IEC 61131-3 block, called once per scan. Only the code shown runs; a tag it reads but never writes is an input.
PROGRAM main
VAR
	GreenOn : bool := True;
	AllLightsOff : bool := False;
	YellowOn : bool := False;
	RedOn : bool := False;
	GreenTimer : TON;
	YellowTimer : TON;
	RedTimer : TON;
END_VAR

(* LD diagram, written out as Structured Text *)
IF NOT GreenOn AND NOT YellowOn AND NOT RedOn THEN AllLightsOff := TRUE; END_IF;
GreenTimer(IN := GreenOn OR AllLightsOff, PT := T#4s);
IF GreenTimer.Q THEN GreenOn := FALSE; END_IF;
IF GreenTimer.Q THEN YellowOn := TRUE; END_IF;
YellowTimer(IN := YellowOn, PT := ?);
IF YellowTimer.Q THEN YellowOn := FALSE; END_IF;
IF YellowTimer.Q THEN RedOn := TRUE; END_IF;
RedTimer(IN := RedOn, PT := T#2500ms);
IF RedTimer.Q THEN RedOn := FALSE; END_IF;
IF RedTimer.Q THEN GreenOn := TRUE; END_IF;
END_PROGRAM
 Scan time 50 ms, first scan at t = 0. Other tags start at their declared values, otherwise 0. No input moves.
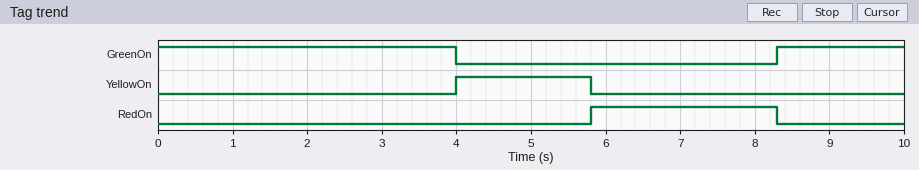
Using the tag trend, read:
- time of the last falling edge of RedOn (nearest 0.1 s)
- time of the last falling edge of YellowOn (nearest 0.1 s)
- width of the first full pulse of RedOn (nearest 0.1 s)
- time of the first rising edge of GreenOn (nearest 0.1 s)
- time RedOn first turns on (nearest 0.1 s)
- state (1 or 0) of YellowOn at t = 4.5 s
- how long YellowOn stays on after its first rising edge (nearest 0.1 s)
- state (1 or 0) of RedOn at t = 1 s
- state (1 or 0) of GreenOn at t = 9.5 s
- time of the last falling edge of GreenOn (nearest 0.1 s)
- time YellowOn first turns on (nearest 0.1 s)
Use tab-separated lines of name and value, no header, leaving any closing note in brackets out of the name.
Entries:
time of the last falling edge of RedOn	8.3 s
time of the last falling edge of YellowOn	5.8 s
width of the first full pulse of RedOn	2.5 s
time of the first rising edge of GreenOn	8.3 s
time RedOn first turns on	5.8 s
state (1 or 0) of YellowOn at t = 4.5 s	1
how long YellowOn stays on after its first rising edge	1.8 s
state (1 or 0) of RedOn at t = 1 s	0
state (1 or 0) of GreenOn at t = 9.5 s	1
time of the last falling edge of GreenOn	4.0 s
time YellowOn first turns on	4.0 s
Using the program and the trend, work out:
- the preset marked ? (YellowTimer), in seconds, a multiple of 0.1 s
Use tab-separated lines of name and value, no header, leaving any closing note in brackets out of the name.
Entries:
the preset marked ? (YellowTimer), in seconds, a multiple of 0.1 s	1.8 s
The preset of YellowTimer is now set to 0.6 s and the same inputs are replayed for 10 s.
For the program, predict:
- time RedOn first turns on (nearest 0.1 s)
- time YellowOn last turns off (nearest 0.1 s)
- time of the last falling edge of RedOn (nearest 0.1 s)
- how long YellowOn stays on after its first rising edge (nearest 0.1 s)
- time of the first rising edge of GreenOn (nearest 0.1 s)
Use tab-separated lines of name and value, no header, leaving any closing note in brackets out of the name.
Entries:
time RedOn first turns on	4.6 s
time YellowOn last turns off	4.6 s
time of the last falling edge of RedOn	7.1 s
how long YellowOn stays on after its first rising edge	0.6 s
time of the first rising edge of GreenOn	7.1 s
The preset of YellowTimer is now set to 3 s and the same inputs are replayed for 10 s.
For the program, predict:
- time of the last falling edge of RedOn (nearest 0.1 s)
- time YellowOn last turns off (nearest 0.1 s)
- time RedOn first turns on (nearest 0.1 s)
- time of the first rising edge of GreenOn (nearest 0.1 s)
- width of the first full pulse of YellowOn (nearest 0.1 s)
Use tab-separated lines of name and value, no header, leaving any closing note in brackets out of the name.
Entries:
time of the last falling edge of RedOn	9.5 s
time YellowOn last turns off	7.0 s
time RedOn first turns on	7.0 s
time of the first rising edge of GreenOn	9.5 s
width of the first full pulse of YellowOn	3.0 s
